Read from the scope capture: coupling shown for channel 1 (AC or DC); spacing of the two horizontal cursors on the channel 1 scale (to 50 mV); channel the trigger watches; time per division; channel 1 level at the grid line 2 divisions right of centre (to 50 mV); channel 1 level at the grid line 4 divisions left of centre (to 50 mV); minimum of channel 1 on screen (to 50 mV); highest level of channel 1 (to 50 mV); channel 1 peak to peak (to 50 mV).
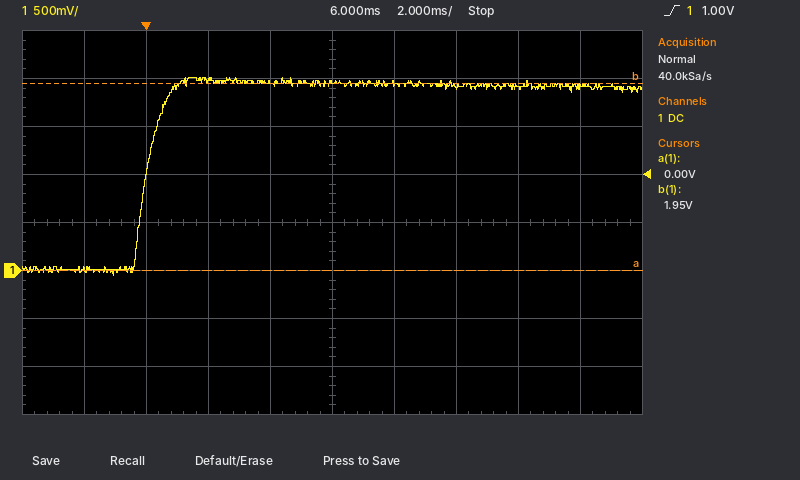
DC
1.95 V
channel 1
2 ms
1.90 V
0 mV
-50 mV
2.00 V
2.05 V
